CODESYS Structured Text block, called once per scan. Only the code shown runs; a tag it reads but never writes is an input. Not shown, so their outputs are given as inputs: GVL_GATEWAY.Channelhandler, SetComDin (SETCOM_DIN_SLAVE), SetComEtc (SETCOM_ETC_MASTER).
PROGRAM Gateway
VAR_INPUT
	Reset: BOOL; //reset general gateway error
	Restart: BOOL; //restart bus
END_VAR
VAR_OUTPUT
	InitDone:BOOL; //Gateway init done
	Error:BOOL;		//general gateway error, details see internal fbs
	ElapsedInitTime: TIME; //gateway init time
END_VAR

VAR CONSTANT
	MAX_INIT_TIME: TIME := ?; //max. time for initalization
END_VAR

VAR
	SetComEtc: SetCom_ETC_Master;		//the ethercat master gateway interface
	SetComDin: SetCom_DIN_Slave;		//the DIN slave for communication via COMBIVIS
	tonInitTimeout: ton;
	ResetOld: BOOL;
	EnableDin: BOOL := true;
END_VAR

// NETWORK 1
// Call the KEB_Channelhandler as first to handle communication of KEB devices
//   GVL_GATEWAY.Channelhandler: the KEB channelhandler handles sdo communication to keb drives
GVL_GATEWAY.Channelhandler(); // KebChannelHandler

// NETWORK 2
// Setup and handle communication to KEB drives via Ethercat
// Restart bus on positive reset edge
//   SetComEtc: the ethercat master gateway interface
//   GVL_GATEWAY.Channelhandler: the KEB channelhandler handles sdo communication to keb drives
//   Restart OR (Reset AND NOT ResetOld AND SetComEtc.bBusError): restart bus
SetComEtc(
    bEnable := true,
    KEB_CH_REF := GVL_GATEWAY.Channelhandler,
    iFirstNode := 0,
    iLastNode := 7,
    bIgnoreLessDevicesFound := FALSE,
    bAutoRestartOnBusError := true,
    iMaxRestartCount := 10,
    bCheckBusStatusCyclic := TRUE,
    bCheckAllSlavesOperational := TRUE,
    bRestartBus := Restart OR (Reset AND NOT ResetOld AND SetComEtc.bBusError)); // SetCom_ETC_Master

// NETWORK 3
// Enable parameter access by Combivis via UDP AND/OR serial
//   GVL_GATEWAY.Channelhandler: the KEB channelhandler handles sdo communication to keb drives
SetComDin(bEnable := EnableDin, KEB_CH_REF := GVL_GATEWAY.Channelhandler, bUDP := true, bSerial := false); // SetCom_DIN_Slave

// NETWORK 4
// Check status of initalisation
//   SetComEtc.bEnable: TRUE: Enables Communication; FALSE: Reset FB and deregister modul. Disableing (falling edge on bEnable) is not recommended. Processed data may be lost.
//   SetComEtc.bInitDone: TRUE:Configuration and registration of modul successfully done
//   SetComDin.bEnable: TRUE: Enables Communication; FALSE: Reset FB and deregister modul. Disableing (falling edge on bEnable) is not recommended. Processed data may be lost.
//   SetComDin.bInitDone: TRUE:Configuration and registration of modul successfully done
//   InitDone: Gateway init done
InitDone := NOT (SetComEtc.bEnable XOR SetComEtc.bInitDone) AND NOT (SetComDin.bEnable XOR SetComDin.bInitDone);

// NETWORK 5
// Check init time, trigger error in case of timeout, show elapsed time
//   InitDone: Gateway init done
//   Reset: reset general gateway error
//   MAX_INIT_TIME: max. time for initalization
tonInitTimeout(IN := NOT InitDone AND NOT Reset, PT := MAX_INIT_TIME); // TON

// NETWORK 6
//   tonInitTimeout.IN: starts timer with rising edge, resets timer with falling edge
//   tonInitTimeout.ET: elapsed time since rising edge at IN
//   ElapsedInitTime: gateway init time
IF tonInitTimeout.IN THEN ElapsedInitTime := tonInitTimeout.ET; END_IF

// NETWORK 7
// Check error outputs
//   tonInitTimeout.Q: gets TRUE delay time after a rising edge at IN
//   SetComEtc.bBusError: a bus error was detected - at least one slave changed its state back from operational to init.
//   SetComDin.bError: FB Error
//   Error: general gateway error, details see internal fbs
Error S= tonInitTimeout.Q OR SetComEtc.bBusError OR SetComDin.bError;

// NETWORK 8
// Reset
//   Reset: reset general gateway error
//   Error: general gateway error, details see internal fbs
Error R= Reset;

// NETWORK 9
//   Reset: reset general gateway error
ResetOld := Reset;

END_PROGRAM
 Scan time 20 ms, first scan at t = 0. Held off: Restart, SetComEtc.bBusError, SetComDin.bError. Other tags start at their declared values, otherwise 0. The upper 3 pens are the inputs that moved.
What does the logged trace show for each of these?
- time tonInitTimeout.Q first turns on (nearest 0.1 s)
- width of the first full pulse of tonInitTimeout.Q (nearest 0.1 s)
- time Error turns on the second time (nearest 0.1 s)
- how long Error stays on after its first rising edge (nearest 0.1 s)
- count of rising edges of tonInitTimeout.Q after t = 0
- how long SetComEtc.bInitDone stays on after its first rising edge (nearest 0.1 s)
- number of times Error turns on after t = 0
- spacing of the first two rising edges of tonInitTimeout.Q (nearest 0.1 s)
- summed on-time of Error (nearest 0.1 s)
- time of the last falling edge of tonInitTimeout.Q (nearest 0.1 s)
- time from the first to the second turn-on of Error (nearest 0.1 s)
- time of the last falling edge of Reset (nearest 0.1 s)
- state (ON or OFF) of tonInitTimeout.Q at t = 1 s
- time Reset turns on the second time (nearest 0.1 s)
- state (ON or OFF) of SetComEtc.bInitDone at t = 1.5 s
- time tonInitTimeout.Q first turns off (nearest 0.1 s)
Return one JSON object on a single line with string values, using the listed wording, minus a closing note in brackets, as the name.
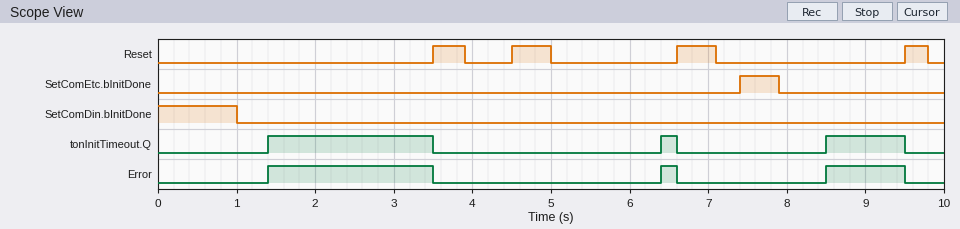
{"time tonInitTimeout.Q first turns on": "1.4 s", "width of the first full pulse of tonInitTimeout.Q": "2.1 s", "time Error turns on the second time": "6.4 s", "how long Error stays on after its first rising edge": "2.1 s", "count of rising edges of tonInitTimeout.Q after t = 0": "3", "how long SetComEtc.bInitDone stays on after its first rising edge": "0.5 s", "number of times Error turns on after t = 0": "3", "spacing of the first two rising edges of tonInitTimeout.Q": "5.0 s", "summed on-time of Error": "3.3 s", "time of the last falling edge of tonInitTimeout.Q": "9.5 s", "time from the first to the second turn-on of Error": "5.0 s", "time of the last falling edge of Reset": "9.8 s", "state (ON or OFF) of tonInitTimeout.Q at t = 1 s": "OFF", "time Reset turns on the second time": "4.5 s", "state (ON or OFF) of SetComEtc.bInitDone at t = 1.5 s": "OFF", "time tonInitTimeout.Q first turns off": "3.5 s"}
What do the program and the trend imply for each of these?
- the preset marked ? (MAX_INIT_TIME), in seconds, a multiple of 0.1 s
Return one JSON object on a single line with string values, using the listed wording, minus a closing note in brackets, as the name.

{"the preset marked ? (MAX_INIT_TIME), in seconds, a multiple of 0.1 s": "1.4 s"}
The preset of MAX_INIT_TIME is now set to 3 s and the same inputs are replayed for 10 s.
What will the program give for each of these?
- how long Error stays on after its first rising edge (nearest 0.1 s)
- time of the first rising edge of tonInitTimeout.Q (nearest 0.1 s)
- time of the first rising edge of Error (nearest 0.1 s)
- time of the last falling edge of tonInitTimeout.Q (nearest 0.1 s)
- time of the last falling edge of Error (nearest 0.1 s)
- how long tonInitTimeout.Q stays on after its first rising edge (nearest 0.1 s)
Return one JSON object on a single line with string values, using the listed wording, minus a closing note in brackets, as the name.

{"how long Error stays on after its first rising edge": "0.5 s", "time of the first rising edge of tonInitTimeout.Q": "3.0 s", "time of the first rising edge of Error": "3.0 s", "time of the last falling edge of tonInitTimeout.Q": "3.5 s", "time of the last falling edge of Error": "3.5 s", "how long tonInitTimeout.Q stays on after its first rising edge": "0.5 s"}
